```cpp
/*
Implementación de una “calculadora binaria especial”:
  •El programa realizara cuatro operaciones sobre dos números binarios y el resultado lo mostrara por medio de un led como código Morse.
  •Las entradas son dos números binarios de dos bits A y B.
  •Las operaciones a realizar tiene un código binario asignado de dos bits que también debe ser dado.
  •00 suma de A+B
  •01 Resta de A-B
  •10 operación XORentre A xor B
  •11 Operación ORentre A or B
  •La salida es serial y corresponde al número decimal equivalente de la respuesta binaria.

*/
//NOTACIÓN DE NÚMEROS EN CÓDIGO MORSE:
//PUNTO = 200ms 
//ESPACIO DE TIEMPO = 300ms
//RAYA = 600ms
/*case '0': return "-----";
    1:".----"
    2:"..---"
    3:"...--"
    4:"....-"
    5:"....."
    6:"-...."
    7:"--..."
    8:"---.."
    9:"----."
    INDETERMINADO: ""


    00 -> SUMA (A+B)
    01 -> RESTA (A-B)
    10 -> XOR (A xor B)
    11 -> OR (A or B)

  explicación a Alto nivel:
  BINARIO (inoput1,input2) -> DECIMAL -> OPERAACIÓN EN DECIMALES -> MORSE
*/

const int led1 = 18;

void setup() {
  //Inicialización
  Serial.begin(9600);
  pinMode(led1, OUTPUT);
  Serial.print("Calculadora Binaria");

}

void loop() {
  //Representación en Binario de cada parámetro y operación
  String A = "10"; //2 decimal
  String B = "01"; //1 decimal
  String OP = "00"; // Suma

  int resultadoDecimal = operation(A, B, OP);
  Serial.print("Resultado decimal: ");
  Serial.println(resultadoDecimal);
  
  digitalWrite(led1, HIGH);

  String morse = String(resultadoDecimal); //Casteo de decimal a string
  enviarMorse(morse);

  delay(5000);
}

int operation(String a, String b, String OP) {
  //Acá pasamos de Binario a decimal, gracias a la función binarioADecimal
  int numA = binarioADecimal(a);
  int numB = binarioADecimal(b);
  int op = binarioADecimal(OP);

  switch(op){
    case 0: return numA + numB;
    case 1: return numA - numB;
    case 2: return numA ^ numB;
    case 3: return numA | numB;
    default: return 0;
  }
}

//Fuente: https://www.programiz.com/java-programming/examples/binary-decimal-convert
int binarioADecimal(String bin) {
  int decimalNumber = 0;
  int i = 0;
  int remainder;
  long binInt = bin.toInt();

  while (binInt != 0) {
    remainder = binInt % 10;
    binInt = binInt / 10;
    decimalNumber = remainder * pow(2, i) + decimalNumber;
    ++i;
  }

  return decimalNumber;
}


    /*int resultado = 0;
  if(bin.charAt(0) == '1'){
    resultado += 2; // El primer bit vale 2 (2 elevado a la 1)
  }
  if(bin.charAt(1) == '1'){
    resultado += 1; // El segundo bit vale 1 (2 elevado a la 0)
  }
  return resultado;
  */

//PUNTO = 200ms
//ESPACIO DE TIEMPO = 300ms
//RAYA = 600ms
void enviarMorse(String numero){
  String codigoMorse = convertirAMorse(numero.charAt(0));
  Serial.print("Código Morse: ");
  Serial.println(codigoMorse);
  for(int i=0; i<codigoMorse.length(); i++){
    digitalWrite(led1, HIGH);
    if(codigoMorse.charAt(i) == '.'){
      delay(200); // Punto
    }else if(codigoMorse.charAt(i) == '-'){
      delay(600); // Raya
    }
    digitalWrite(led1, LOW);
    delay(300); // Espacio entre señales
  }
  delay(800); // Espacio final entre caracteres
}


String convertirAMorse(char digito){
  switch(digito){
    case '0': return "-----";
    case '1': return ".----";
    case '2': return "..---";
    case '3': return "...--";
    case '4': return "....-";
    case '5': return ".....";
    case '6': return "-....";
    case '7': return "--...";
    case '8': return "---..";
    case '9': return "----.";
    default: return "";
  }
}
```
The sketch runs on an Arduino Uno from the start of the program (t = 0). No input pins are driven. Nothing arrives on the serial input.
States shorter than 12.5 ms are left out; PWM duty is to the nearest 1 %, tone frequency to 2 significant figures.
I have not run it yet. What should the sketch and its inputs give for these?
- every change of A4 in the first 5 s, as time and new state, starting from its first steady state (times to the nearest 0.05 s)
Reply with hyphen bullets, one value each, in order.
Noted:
- 0 s high; 0.2 s low; 0.5 s high; 0.7 s low; 1 s high; 1.2 s low; 1.5 s high; 2.1 s low; 2.4 s high; 3 s low
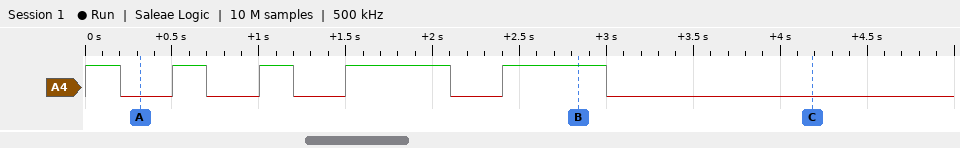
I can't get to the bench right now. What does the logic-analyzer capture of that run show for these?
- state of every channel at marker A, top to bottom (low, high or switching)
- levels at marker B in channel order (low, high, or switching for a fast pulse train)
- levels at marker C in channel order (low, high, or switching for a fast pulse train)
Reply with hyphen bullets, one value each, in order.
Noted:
- A4 low
- A4 high
- A4 low
